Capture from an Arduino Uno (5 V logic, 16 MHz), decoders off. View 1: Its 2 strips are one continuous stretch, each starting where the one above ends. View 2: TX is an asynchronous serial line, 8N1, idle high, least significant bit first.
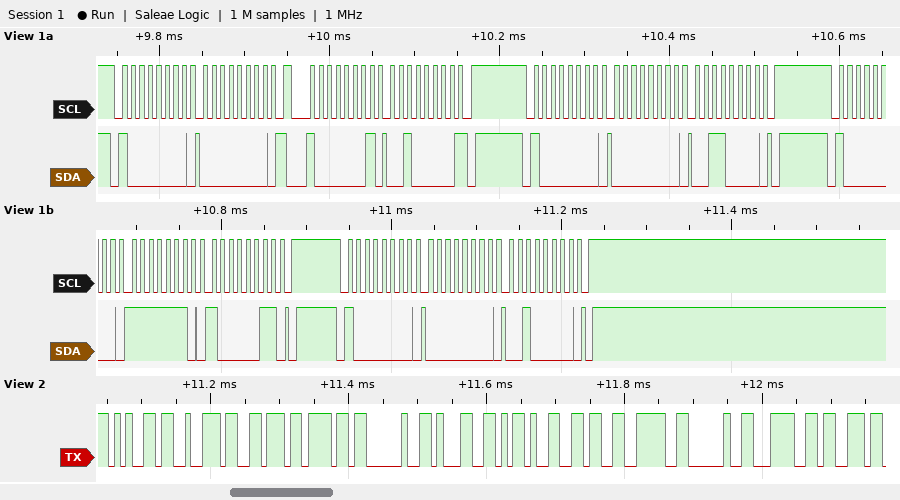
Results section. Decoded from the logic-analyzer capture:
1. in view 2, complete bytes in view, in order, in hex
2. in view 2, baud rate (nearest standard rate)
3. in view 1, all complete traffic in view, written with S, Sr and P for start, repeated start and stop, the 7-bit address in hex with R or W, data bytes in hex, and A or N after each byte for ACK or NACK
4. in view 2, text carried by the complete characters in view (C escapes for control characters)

0x65 0x72 0x76 0x6F 0x20 0x31 0x2D 0x36 0x3E 0x20 0x3C 0x73
115200 baud
S 40W A 00 A Sr 40R A 20 N P S 40W A 00 A 30 A P S 40W A FE A 83 A P S 40W A 00 A 20 A P
"ervo 1-6> <s"
